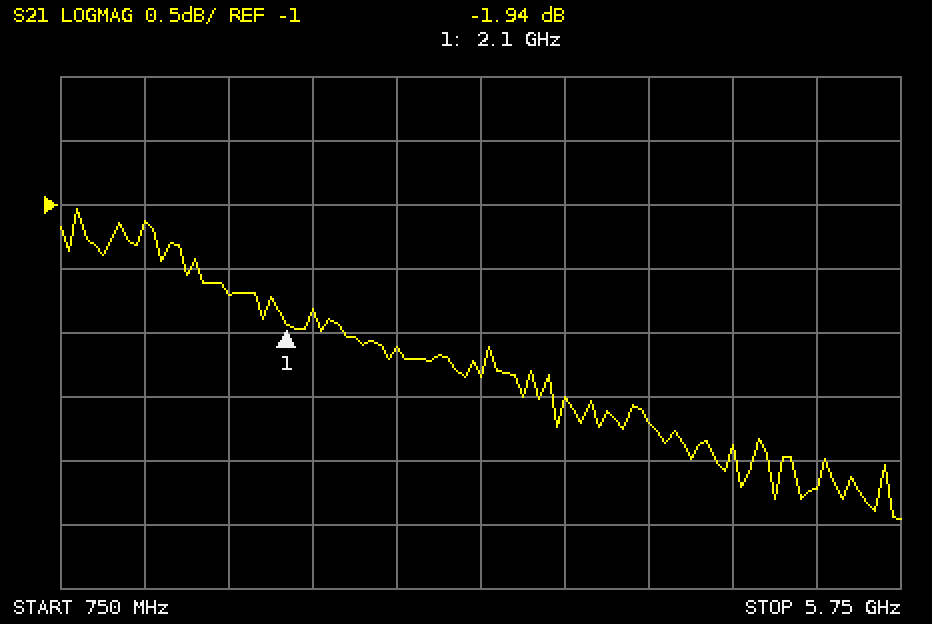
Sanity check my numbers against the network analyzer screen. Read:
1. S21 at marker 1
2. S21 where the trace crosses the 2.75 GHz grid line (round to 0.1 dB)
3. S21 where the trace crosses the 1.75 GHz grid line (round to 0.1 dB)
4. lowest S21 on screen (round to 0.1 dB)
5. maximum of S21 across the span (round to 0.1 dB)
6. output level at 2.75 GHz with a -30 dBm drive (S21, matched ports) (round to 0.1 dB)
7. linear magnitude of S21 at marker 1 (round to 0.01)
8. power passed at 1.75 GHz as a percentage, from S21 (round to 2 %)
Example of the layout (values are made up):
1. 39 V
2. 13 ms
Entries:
1. -1.94 dB
2. -2.1 dB
3. -1.7 dB
4. -3.5 dB
5. -1.0 dB
6. -32.1 dBm
7. 0.80
8. 68 %
